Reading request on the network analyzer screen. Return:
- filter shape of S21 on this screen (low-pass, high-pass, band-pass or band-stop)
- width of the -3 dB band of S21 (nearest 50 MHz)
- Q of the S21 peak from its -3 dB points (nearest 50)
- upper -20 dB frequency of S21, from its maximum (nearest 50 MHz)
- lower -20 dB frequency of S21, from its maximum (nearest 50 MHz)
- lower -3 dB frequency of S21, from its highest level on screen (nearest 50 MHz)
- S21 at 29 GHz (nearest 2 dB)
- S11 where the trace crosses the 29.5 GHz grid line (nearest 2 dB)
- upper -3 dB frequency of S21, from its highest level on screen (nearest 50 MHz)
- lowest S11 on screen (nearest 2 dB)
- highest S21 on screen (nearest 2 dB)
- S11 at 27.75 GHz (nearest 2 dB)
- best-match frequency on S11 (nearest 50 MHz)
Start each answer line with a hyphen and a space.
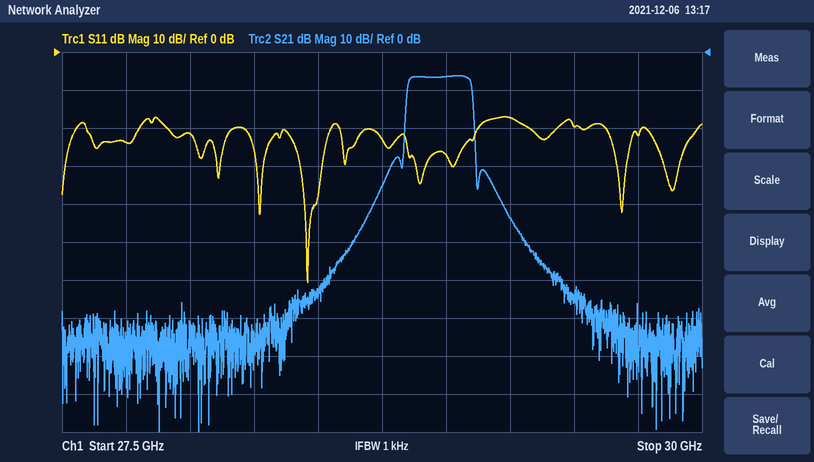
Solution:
- band-pass
- 250 MHz
- 100
- 29.10 GHz
- 28.85 GHz
- 28.85 GHz
- -6 dB
- -20 dB
- 29.10 GHz
- -60 dB
- -6 dB
- -24 dB
- 28.45 GHz
